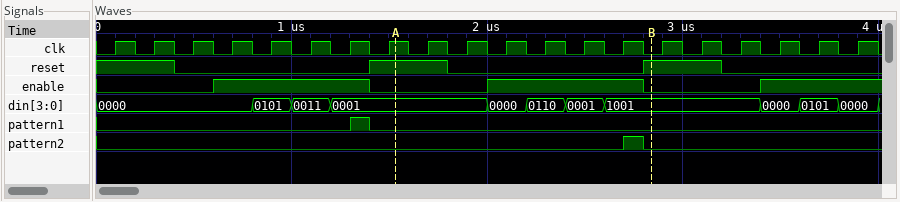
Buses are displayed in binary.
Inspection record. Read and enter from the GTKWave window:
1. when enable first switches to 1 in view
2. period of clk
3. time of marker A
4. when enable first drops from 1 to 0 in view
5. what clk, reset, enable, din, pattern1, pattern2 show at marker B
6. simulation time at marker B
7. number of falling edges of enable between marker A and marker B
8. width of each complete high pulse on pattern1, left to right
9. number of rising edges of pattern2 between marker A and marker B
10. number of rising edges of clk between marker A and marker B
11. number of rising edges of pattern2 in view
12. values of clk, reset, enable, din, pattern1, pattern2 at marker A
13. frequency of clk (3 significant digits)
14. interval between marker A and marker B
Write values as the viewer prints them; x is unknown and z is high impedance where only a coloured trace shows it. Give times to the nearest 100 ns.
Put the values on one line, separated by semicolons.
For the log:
600 ns; 200 ns; 1500 ns; 1400 ns; clk=0, reset=1, enable=0, din=1001, pattern1=0, pattern2=0; 2800 ns; 1; 100 ns; 1; 6; 1; clk=1, reset=1, enable=0, din=0001, pattern1=0, pattern2=0; 5.00 MHz; 1300 ns
